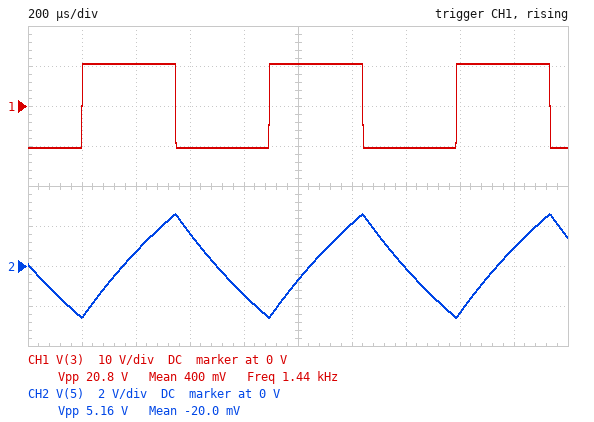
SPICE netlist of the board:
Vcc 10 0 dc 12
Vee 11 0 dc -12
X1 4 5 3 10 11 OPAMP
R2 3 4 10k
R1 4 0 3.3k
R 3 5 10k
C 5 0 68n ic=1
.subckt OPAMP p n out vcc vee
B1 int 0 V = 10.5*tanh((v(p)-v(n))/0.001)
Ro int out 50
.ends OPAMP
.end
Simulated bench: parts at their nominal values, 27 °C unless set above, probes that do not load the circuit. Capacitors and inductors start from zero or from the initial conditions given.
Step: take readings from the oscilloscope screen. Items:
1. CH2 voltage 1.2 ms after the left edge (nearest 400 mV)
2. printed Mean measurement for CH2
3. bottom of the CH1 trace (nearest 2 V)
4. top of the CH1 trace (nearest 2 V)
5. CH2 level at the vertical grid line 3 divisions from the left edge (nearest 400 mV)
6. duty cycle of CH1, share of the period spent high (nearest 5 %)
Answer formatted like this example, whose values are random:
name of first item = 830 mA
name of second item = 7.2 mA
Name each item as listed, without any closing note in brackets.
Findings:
CH2 voltage 1.2 ms after the left edge = 2.0 V
printed Mean measurement for CH2 = -20.0 mV
bottom of the CH1 trace = -10 V
top of the CH1 trace = 10 V
CH2 level at the vertical grid line 3 divisions from the left edge = 1.6 V
duty cycle of CH1, share of the period spent high = 50 %
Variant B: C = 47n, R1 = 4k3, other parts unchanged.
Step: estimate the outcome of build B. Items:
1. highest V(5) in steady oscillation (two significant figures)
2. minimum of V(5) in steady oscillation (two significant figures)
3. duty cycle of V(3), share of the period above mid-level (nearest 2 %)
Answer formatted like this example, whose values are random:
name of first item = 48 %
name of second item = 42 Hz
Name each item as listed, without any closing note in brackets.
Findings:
highest V(5) in steady oscillation = 3.1 V
minimum of V(5) in steady oscillation = -3.1 V
duty cycle of V(3), share of the period above mid-level = 50 %
